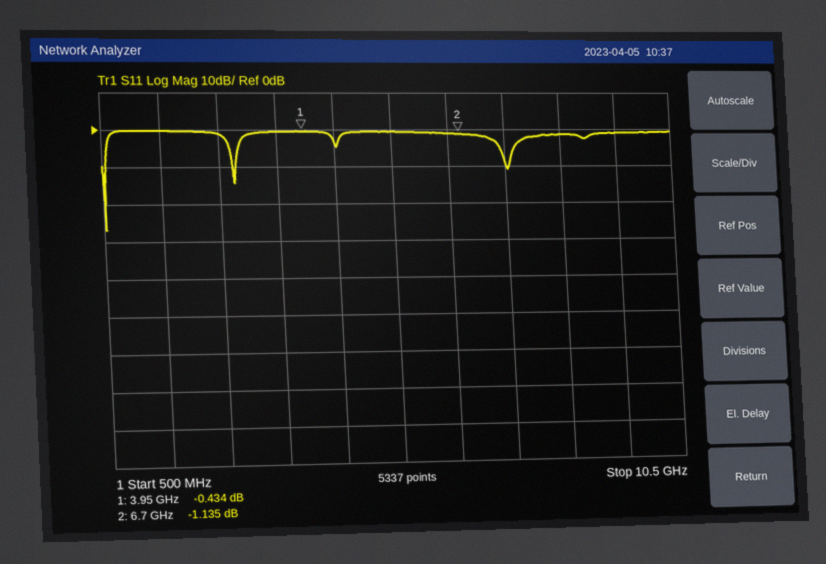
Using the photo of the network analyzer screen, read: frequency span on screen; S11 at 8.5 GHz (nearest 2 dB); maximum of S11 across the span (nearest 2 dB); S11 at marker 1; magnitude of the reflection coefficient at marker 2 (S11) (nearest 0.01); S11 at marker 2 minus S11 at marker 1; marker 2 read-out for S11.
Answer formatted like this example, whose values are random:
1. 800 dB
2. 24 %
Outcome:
1. 10 GHz
2. -2 dB
3. 0 dB
4. -0.434 dB
5. 0.88
6. -0.701 dB
7. -1.135 dB
